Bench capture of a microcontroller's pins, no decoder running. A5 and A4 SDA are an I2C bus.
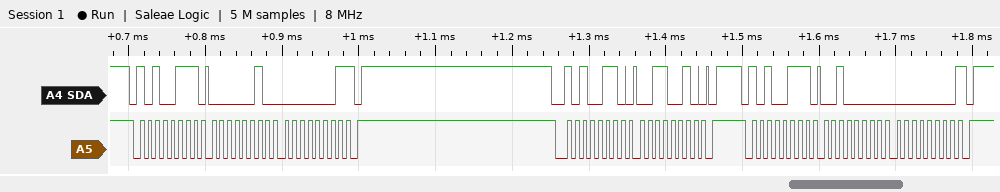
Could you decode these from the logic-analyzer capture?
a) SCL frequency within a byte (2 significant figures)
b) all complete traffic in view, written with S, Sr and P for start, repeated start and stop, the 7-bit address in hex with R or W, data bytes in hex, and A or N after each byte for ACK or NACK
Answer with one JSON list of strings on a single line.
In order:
["100 kHz", "S 53R A 02 A 01 N P S 53W A 32 A P S 53R A 20 A 00 N P"]
